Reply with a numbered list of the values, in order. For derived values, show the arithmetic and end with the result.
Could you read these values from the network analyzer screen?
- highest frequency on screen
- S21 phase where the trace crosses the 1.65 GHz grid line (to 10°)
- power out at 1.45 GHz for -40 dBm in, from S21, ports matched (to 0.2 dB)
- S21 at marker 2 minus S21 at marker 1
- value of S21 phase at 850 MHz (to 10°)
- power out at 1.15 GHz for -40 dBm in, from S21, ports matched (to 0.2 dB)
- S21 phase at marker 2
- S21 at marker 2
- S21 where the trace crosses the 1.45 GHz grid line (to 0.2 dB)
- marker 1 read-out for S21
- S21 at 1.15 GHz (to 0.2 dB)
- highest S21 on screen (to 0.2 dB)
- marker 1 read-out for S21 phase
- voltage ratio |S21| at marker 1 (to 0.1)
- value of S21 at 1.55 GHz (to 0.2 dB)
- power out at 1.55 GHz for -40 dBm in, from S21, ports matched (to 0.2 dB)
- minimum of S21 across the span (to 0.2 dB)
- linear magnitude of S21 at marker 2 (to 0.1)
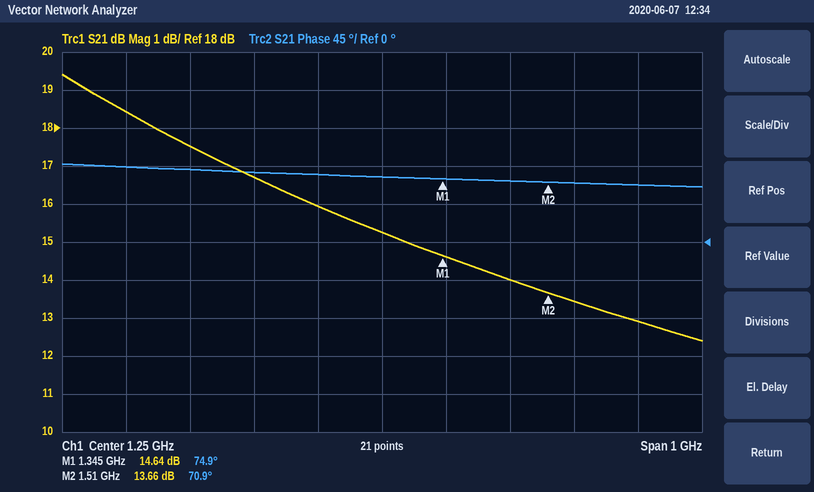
1. 1.75 GHz
2. 70°
3. -40 dBm + (14.0 dB) = -26.0 dBm
4. 13.66 − (14.64) = -0.98 dB
5. 90°
6. -40 dBm + (16.0 dB) = -24.0 dBm
7. 70.9°
8. 13.66 dB
9. 14.0 dB
10. 14.64 dB
11. 16.0 dB
12. 19.4 dB
13. 74.9°
14. 10^(14.64/20) ≈ 5.4
15. 13.4 dB
16. -40 dBm + (13.4 dB) = -26.6 dBm
17. 12.4 dB
18. 10^(13.66/20) ≈ 4.8
